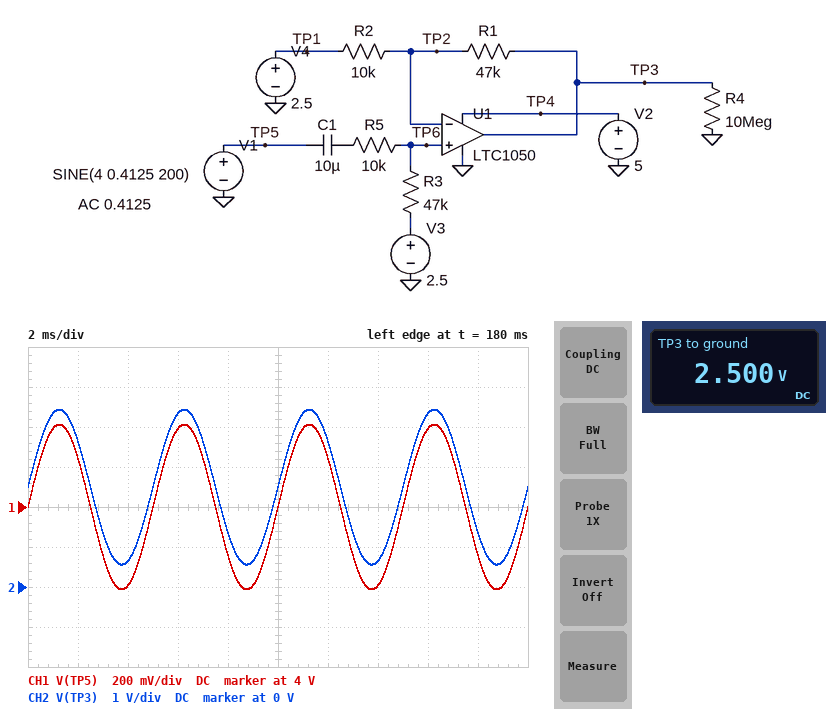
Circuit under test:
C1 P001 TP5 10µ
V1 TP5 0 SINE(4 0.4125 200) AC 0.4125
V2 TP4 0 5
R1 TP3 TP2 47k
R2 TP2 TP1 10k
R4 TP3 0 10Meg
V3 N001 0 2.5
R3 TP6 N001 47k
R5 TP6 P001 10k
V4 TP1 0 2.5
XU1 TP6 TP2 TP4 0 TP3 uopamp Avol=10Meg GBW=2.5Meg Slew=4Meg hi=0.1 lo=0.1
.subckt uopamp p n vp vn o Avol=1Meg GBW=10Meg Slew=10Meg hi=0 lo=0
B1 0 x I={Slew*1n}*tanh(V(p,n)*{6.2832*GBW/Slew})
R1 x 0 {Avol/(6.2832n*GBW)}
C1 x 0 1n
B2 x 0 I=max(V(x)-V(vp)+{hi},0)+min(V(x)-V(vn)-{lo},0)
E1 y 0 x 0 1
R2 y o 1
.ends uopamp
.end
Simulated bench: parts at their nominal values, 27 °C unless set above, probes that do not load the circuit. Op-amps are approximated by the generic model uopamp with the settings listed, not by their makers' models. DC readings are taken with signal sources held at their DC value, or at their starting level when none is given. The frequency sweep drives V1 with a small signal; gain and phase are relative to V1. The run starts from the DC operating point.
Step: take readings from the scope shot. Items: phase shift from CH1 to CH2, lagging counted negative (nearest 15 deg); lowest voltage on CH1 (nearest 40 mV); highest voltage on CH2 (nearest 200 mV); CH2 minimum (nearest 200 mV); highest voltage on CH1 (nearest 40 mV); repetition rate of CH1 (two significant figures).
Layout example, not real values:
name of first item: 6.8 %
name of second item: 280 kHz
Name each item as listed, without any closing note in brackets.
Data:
phase shift from CH1 to CH2, lagging counted negative: 0 deg
lowest voltage on CH1: 3.60 V
highest voltage on CH2: 4.4 V
CH2 minimum: 600 mV
highest voltage on CH1: 4.40 V
repetition rate of CH1: 200 Hz
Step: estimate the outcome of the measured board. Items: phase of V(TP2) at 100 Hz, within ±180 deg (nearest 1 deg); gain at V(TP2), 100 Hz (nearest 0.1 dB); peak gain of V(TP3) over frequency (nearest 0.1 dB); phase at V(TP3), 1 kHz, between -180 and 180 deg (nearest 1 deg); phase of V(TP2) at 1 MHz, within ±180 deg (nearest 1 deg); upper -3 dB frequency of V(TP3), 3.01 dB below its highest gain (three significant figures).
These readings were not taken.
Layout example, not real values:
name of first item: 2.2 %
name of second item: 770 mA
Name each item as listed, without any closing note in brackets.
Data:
phase of V(TP2) at 100 Hz, within ±180 deg: 0 deg
gain at V(TP2), 100 Hz: -1.7 dB
peak gain of V(TP3) over frequency: 13.4 dB
phase at V(TP3), 1 kHz, between -180 and 180 deg: 0 deg
phase of V(TP2) at 1 MHz, within ±180 deg: -66 deg
upper -3 dB frequency of V(TP3), 3.01 dB below its highest gain: 439 kHz
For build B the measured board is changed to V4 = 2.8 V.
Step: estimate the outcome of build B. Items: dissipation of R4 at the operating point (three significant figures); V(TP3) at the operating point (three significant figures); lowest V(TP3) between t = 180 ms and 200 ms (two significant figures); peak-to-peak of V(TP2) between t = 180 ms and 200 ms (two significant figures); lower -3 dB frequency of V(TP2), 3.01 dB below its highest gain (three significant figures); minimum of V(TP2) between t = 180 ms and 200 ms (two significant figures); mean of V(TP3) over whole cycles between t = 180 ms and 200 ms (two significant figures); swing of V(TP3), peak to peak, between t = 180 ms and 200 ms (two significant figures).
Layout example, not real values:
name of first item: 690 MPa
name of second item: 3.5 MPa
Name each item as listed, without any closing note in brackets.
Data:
dissipation of R4 at the operating point: 119 nW
V(TP3) at the operating point: 1.09 V
lowest V(TP3) between t = 180 ms and 200 ms: 98 mV
peak-to-peak of V(TP2) between t = 180 ms and 200 ms: 510 mV
lower -3 dB frequency of V(TP2), 3.01 dB below its highest gain: 279 mHz
minimum of V(TP2) between t = 180 ms and 200 ms: 2.3 V
mean of V(TP3) over whole cycles between t = 180 ms and 200 ms: 1.3 V
swing of V(TP3), peak to peak, between t = 180 ms and 200 ms: 2.9 V
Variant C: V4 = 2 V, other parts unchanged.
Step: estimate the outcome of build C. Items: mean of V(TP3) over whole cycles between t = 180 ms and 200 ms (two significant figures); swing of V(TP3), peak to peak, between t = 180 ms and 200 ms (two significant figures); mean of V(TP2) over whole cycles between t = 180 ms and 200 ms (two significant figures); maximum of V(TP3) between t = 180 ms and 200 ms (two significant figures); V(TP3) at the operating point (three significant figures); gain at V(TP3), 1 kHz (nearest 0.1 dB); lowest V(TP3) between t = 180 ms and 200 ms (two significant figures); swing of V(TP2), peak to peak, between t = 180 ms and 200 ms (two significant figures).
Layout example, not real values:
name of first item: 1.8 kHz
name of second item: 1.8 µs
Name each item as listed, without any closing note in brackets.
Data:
mean of V(TP3) over whole cycles between t = 180 ms and 200 ms: 4.3 V
swing of V(TP3), peak to peak, between t = 180 ms and 200 ms: 2.0 V
mean of V(TP2) over whole cycles between t = 180 ms and 200 ms: 2.4 V
maximum of V(TP3) between t = 180 ms and 200 ms: 4.9 V
V(TP3) at the operating point: 4.85 V
gain at V(TP3), 1 kHz: 13.4 dB
lowest V(TP3) between t = 180 ms and 200 ms: 2.9 V
swing of V(TP2), peak to peak, between t = 180 ms and 200 ms: 350 mV
